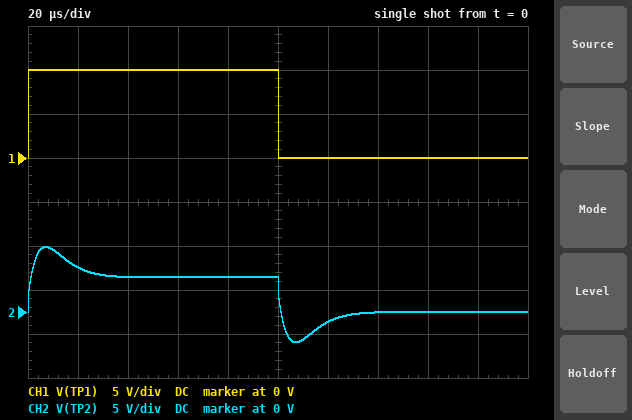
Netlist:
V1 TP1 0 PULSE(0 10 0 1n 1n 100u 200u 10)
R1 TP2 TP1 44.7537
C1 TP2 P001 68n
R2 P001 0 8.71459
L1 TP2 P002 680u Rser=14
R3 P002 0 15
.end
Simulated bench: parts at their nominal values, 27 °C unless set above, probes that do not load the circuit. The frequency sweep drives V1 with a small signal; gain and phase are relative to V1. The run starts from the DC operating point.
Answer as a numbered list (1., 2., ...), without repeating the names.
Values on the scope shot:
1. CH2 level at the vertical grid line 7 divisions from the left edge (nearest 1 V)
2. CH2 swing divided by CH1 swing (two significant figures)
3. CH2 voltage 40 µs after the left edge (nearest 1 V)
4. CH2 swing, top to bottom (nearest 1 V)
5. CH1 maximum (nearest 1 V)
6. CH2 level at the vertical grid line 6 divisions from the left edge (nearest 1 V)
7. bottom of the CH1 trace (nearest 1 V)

1. 0 V
2. 1.1
3. 4 V
4. 11 V
5. 10 V
6. -1 V
7. 0 V
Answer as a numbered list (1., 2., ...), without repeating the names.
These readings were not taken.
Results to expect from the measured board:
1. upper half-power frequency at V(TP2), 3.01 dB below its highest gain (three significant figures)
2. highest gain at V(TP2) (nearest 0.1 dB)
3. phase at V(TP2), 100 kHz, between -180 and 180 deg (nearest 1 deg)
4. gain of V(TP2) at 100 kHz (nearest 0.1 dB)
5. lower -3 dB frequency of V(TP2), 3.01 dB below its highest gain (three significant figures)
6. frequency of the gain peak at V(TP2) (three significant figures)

1. 63.8 kHz
2. -1.2 dB
3. -44 deg
4. -7.1 dB
5. 9.43 kHz
6. 26.2 kHz
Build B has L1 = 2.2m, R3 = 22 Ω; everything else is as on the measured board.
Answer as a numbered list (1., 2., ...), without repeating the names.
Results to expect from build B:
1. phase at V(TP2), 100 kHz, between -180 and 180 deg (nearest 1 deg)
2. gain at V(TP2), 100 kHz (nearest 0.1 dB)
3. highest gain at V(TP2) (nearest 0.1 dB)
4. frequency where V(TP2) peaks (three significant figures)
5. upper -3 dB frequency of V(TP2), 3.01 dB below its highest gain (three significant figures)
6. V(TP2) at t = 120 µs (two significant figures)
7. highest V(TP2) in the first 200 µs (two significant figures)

1. -45 deg
2. -7.3 dB
3. -0.5 dB
4. 15.1 kHz
5. 52.2 kHz
6. -3.2 V
7. 8.6 V
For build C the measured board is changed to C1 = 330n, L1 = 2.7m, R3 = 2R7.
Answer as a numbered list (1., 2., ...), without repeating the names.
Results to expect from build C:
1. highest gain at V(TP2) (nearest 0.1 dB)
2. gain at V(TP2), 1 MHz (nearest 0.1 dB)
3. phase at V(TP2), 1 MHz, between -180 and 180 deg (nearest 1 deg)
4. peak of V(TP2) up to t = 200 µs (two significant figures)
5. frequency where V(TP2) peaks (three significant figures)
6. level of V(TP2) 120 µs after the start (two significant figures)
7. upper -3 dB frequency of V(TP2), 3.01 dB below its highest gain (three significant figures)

1. -1.1 dB
2. -15.7 dB
3. -3 deg
4. 7.1 V
5. 5.62 kHz
6. -3.3 V
7. 13.1 kHz
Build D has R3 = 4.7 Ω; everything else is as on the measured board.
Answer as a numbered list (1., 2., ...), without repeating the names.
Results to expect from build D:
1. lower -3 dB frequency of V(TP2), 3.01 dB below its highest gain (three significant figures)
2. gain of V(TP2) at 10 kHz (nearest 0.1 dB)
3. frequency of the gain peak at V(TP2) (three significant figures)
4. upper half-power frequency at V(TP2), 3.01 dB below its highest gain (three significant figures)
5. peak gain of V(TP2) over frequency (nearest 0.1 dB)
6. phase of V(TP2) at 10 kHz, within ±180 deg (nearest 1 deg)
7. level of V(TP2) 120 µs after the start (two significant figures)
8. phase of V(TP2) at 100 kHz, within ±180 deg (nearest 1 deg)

1. 9.71 kHz
2. -3.8 dB
3. 25.0 kHz
4. 61.3 kHz
5. -1.0 dB
6. 26 deg
7. -1.6 V
8. -44 deg
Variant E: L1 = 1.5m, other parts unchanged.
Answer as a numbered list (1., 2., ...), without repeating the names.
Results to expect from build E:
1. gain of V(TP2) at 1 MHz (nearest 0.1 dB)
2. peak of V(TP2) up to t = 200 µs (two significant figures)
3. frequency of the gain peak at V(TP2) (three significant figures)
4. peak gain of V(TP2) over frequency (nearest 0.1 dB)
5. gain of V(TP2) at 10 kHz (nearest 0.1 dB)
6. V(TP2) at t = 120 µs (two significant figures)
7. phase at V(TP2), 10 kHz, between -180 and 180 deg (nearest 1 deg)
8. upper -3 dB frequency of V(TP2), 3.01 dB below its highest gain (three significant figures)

1. -15.5 dB
2. 8.2 V
3. 17.8 kHz
4. -0.6 dB
5. -1.3 dB
6. -2.9 V
7. 12 deg
8. 54.4 kHz
